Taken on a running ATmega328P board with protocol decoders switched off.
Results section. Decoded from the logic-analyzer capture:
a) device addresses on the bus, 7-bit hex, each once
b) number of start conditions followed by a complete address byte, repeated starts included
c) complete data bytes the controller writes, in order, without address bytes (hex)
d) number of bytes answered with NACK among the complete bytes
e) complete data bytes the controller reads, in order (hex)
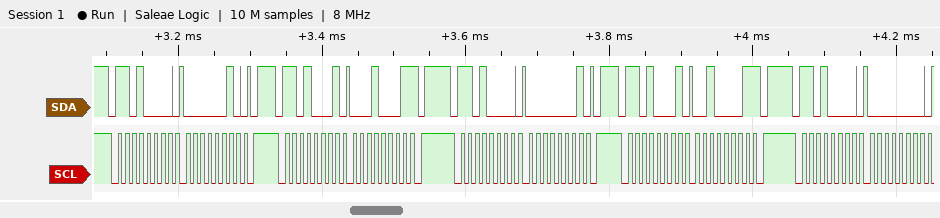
0x68
5
02 01 00
2
11 21
